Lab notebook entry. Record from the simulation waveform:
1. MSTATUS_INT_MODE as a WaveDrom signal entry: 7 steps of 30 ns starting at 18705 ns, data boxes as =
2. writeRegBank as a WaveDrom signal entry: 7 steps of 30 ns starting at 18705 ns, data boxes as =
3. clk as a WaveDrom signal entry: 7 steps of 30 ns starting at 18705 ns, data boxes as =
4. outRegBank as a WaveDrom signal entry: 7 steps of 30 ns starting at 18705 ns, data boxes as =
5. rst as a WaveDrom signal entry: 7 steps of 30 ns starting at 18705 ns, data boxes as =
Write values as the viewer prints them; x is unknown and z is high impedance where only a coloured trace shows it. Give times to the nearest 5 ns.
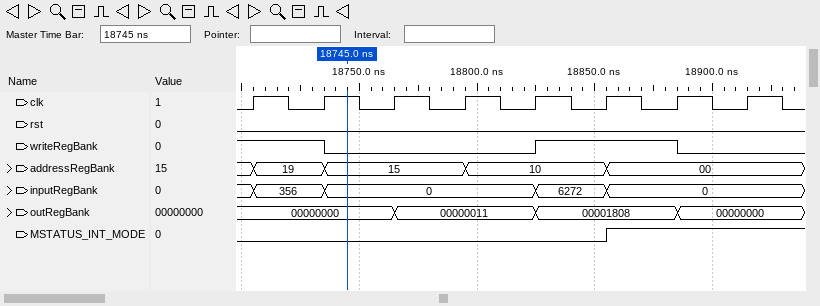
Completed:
{name: 'MSTATUS_INT_MODE', wave: '0....1.'}
{name: 'writeRegBank', wave: '10..1.0'}
{name: 'clk', wave: 'p......'}
{name: 'outRegBank', wave: '=.=.=.=', data: '00000000 00000011 00001808 00000000'}
{name: 'rst', wave: '0......'}
